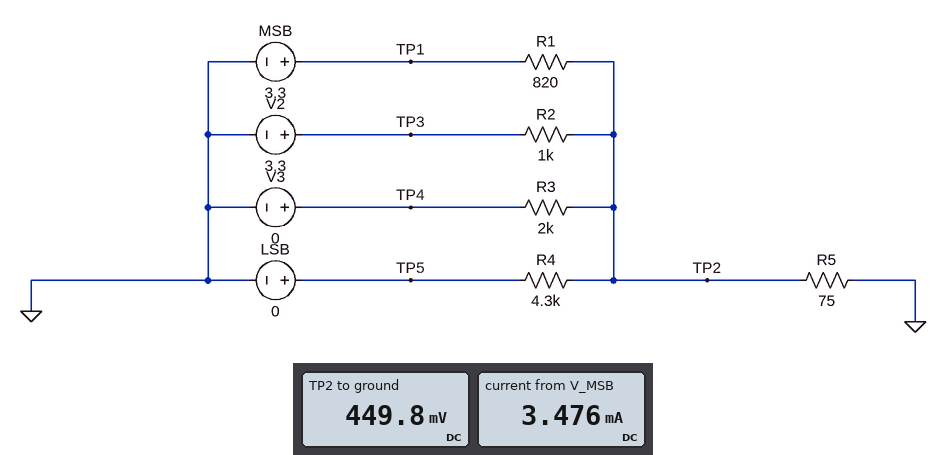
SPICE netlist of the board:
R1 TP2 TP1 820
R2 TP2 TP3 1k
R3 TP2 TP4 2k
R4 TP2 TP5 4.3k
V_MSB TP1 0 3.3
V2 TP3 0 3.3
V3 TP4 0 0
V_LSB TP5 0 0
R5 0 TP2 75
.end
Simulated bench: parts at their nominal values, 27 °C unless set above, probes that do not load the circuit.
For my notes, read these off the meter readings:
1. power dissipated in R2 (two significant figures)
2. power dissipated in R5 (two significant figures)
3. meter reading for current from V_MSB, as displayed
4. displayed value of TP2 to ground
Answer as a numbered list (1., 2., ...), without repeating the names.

1. 8.1 mW
2. 2.7 mW
3. 3.476 mA
4. 449.8 mV
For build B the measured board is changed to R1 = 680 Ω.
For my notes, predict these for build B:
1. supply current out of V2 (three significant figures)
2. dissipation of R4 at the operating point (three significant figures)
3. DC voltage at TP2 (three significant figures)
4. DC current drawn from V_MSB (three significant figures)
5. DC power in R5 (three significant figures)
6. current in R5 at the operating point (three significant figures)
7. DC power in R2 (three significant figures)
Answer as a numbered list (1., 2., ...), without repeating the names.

1. 2.81 mA
2. 56.5 µW
3. 493 mV
4. 4.13 mA
5. 3.24 mW
6. 6.57 mA
7. 7.88 mW
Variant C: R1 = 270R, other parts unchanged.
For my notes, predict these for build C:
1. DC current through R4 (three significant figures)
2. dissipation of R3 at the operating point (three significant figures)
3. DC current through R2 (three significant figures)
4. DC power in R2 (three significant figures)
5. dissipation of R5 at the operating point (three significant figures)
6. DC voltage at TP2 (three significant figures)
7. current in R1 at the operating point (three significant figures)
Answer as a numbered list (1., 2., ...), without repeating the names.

1. 192 µA
2. 342 µW
3. 2.47 mA
4. 6.12 mW
5. 9.12 mW
6. 827 mV
7. 9.16 mA
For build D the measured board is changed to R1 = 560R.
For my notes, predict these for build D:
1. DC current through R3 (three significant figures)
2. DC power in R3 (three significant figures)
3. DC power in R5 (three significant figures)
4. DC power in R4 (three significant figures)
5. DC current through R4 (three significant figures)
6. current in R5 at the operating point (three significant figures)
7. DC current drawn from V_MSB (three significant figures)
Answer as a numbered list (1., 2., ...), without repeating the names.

1. 273 µA
2. 149 µW
3. 3.97 mW
4. 69.2 µW
5. 127 µA
6. 7.27 mA
7. 4.92 mA
